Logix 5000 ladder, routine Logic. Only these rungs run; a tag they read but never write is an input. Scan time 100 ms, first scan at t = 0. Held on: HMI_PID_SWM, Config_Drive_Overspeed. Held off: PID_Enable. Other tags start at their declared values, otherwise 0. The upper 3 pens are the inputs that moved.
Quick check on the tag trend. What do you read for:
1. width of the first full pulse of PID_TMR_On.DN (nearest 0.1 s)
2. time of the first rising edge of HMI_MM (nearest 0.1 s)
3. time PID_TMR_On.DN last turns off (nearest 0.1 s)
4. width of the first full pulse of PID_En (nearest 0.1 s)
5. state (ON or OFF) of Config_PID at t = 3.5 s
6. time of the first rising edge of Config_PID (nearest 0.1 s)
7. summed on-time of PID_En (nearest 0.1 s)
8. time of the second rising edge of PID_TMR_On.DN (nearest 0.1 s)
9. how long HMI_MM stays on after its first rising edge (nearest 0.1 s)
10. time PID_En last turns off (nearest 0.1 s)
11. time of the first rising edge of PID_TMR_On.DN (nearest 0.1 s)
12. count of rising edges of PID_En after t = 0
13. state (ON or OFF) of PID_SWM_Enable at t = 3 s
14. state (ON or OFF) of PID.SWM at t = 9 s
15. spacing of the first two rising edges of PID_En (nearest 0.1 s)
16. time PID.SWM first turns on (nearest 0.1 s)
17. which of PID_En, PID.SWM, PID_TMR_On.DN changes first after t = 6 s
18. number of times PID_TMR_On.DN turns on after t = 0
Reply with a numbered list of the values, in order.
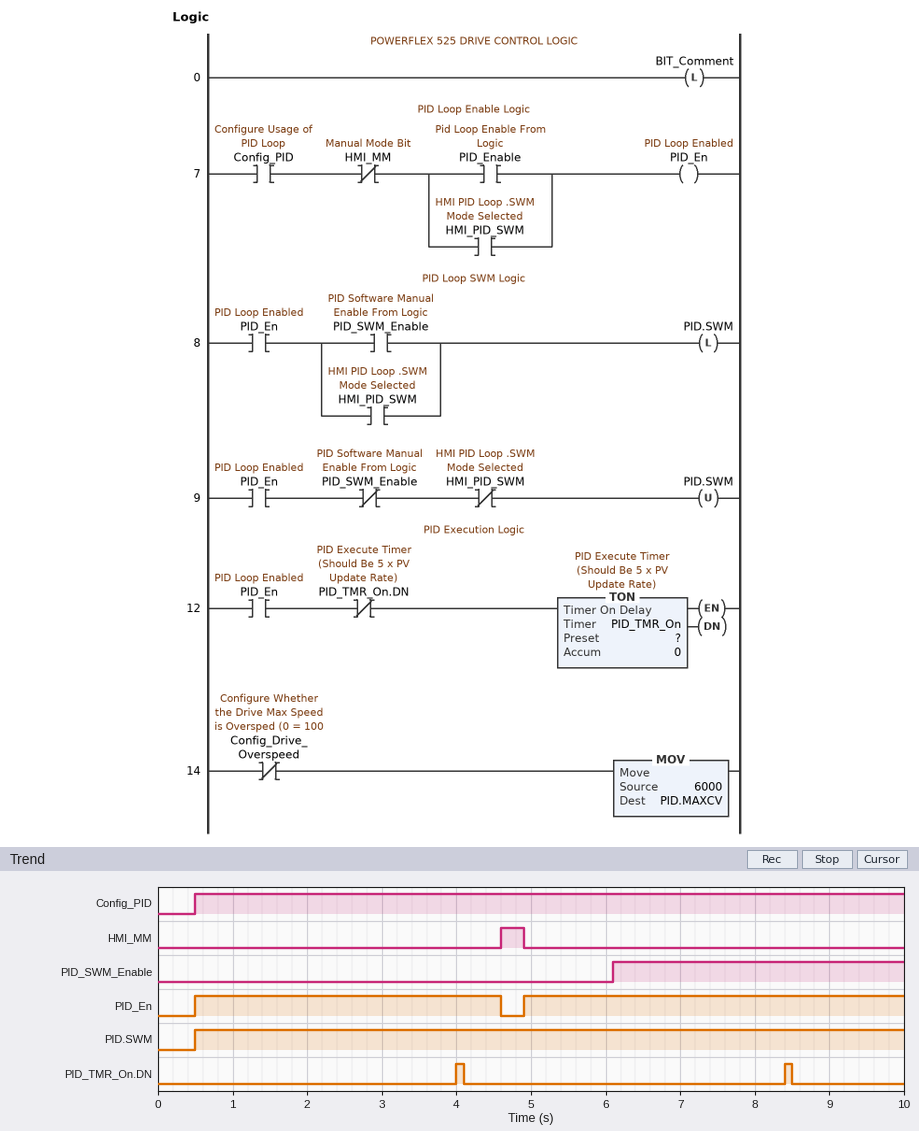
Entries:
1. 0.1 s
2. 4.6 s
3. 8.5 s
4. 4.1 s
5. ON
6. 0.5 s
7. 9.2 s
8. 8.4 s
9. 0.3 s
10. 4.6 s
11. 4.0 s
12. 2
13. OFF
14. ON
15. 4.4 s
16. 0.5 s
17. PID_TMR_On.DN
18. 2
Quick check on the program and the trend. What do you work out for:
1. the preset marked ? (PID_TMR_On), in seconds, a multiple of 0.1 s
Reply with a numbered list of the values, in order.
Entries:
1. 3.5 s
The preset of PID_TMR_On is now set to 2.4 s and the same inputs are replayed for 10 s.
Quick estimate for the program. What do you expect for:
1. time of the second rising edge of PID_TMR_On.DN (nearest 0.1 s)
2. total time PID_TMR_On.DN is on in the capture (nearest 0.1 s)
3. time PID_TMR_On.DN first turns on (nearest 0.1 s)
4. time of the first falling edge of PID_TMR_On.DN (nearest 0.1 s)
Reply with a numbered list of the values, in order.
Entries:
1. 7.3 s
2. 0.3 s
3. 2.9 s
4. 3.0 s
